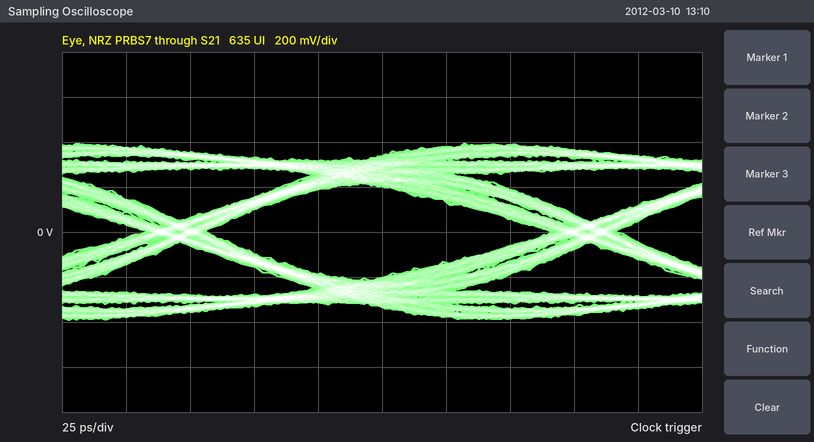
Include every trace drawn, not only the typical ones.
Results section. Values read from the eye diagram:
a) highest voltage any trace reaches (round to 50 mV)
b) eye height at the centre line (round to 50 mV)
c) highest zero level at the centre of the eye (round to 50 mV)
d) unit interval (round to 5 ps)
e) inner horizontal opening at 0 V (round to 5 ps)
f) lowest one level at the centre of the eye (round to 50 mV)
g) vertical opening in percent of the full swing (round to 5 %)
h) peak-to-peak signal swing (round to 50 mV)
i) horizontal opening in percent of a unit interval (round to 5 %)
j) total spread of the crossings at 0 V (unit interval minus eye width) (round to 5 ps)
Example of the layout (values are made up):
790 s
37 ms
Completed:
400 mV
400 mV
-200 mV
160 ps
135 ps
200 mV
50 %
800 mV
85 %
25 ps
